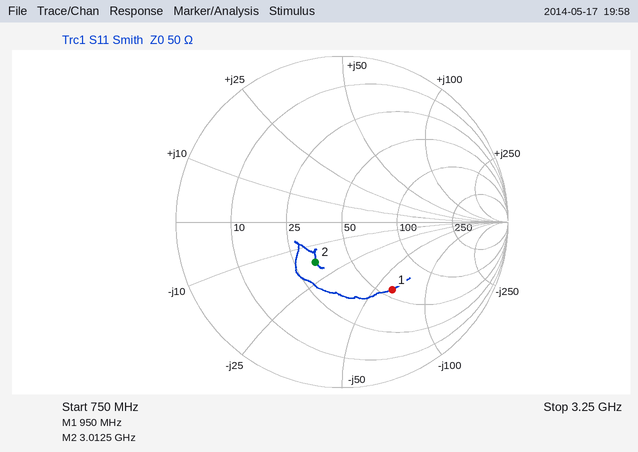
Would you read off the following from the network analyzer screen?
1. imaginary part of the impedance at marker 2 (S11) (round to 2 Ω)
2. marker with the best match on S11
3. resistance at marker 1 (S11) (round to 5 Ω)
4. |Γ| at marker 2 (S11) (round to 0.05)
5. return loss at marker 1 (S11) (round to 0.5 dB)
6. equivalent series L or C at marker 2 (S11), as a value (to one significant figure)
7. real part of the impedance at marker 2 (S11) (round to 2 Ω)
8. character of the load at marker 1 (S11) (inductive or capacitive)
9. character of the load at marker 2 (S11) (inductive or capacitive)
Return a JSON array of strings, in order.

["-18 Ω", "marker 2", "55 Ω", "0.30", "6.0 dB", "3 pF", "32 Ω", "capacitive", "capacitive"]
